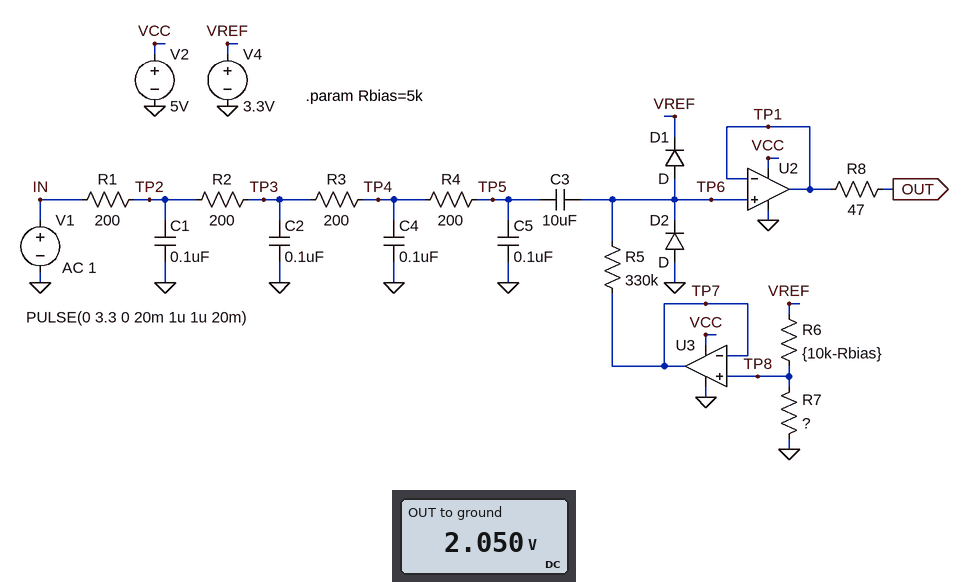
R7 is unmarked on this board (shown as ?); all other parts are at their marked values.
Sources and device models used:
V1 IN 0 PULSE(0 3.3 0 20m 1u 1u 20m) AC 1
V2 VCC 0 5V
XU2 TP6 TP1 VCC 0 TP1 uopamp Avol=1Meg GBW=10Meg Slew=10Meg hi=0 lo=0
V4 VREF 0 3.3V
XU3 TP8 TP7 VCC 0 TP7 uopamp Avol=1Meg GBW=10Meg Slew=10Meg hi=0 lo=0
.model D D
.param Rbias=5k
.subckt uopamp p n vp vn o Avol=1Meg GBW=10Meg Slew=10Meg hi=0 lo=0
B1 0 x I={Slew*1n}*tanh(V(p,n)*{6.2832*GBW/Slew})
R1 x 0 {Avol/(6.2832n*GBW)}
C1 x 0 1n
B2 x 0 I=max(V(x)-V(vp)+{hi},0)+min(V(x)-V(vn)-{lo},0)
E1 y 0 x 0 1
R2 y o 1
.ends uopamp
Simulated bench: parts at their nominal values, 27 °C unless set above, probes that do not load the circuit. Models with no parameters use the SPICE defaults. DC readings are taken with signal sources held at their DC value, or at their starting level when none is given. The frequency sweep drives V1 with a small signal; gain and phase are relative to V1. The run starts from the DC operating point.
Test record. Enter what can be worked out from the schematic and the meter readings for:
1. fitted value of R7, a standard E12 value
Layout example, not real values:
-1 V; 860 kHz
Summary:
8.2 kΩ
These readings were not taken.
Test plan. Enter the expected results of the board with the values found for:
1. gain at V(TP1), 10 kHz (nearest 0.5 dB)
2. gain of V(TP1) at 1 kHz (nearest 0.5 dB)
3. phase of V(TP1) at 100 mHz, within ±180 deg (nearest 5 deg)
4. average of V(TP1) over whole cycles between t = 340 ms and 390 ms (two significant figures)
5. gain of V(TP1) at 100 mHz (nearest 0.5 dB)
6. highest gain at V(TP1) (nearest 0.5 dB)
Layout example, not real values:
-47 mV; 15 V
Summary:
-26.0 dB; -3.5 dB; 25 deg; 2.4 V; -1.0 dB; 0 dB
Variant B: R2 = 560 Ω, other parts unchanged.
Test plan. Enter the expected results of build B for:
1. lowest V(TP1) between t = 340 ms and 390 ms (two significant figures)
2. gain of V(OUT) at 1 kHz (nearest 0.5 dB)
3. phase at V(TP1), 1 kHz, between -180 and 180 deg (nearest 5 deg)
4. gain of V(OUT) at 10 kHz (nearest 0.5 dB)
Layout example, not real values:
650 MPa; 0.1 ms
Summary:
960 mV; -6.0 dB; -75 deg; -31.5 dB
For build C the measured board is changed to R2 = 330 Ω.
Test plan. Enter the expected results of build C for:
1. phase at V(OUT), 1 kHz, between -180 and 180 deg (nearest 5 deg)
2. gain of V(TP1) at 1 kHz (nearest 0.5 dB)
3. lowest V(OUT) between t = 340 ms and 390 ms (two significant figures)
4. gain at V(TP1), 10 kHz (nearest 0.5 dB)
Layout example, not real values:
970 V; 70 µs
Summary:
-65 deg; -4.5 dB; 890 mV; -28.5 dB
